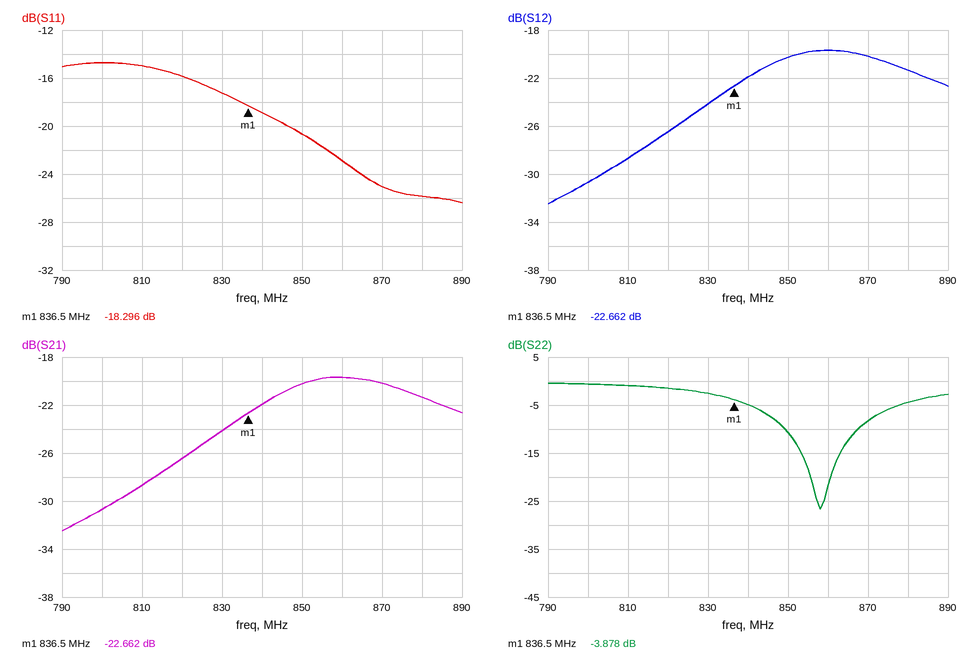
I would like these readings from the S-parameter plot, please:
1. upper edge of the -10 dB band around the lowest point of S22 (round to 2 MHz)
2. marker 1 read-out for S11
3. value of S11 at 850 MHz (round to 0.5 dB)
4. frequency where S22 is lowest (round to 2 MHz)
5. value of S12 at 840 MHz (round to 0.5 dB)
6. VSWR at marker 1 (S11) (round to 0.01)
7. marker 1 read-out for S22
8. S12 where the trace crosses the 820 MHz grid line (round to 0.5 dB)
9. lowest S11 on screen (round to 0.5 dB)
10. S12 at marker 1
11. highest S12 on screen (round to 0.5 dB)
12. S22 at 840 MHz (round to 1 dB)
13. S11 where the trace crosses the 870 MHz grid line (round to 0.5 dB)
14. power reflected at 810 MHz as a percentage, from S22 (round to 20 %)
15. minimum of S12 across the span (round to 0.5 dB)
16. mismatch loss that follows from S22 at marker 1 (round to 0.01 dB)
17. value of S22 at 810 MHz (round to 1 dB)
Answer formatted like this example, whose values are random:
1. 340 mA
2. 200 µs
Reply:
1. 868 MHz
2. -18.296 dB
3. -20.5 dB
4. 858 MHz
5. -22.0 dB
6. 1.28
7. -3.878 dB
8. -26.5 dB
9. -26.5 dB
10. -22.662 dB
11. -19.5 dB
12. -5 dB
13. -25.0 dB
14. 80 %
15. -32.5 dB
16. 2.29 dB
17. -1 dB
